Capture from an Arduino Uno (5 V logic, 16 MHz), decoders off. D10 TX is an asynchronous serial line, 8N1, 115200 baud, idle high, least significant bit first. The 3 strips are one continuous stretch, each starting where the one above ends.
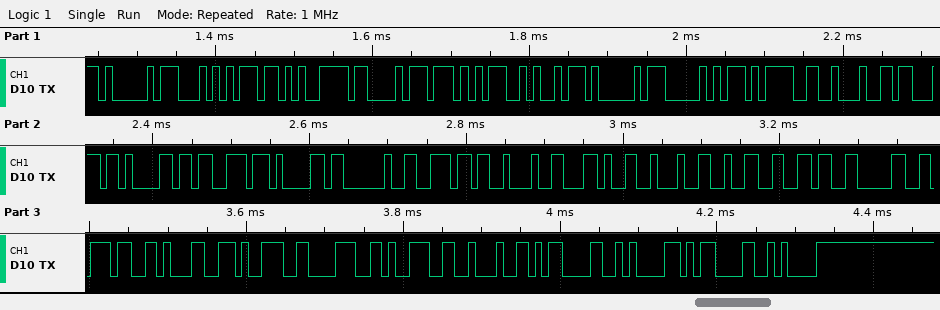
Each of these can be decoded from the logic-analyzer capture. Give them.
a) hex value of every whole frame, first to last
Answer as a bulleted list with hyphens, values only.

- 0x41 0x54 0x2B 0x43 0x57 0x4A 0x41 0x50 0x3D 0x22 0x63 0x61 0x73 0x61 0x20 0x6E 0x22 0x2C 0x22 0x32 0x36 0x30 0x37 0x31 0x39 0x38 0x39 0x22 0x0D 0x0A 0x0D 0x0A
